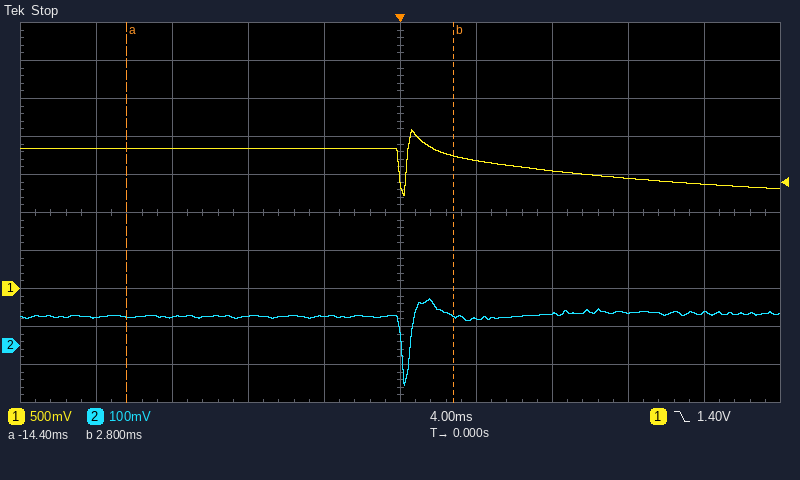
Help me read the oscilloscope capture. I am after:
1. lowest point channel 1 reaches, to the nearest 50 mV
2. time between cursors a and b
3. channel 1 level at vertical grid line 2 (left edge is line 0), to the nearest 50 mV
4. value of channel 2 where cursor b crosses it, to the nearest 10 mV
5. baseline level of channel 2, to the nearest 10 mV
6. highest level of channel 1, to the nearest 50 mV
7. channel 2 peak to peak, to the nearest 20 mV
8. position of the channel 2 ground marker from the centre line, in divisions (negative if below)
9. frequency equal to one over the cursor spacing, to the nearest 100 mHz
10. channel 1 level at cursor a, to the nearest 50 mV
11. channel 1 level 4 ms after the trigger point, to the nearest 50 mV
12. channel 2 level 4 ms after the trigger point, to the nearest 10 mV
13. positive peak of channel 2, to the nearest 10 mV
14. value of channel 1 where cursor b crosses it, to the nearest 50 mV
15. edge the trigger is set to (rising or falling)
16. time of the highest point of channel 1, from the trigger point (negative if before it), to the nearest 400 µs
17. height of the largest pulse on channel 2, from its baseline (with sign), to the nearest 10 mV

1.20 V
17.2 ms
1.85 V
80 mV
80 mV
2.10 V
220 mV
-3.5 div
58.1 Hz
1.85 V
1.70 V
70 mV
120 mV
1.75 V
falling
+800 µs
-180 mV
